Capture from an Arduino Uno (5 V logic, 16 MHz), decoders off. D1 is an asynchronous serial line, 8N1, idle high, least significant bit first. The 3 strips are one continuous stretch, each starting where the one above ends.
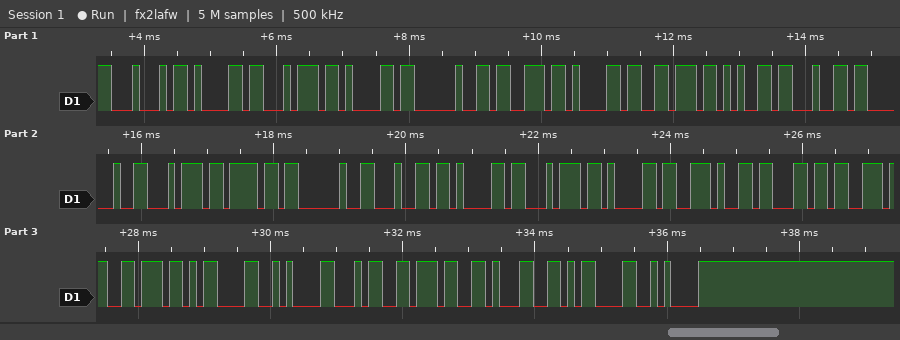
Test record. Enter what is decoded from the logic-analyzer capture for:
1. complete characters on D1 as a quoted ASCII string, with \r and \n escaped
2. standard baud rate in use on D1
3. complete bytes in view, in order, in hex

"Data saved to data.csv\r\n471\r\n"
9600 baud
44 61 74 61 20 73 61 76 65 64 20 74 6F 20 64 61 74 61 2E 63 73 76 0D 0A 34 37 31 0D 0A
